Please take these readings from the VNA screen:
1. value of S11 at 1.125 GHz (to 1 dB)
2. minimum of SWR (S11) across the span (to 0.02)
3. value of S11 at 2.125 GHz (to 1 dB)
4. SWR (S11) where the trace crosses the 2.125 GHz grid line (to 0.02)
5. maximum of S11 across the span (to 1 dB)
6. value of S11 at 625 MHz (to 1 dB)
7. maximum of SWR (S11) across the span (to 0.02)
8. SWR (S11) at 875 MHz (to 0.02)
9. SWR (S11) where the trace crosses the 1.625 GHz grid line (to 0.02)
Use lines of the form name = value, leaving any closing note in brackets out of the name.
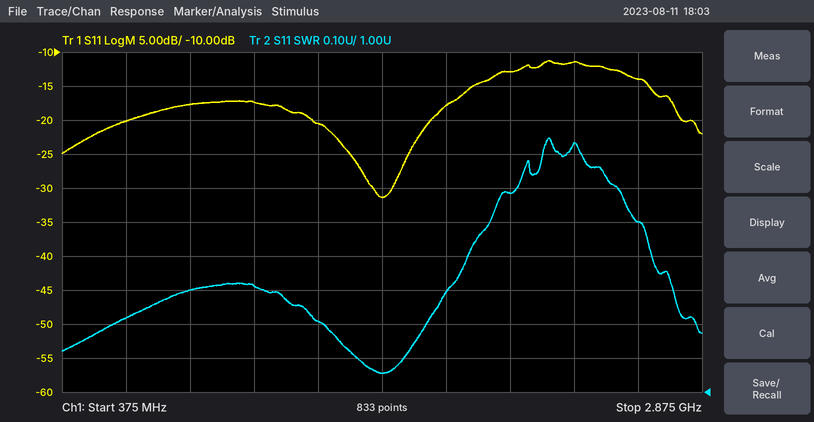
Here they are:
value of S11 at 1.125 GHz = -17 dB
minimum of SWR (S11) across the span = 1.06
value of S11 at 2.125 GHz = -13 dB
SWR (S11) where the trace crosses the 2.125 GHz grid line = 1.58
maximum of S11 across the span = -11 dB
value of S11 at 625 MHz = -20 dB
maximum of SWR (S11) across the span = 1.74
SWR (S11) at 875 MHz = 1.30
SWR (S11) where the trace crosses the 1.625 GHz grid line = 1.06
